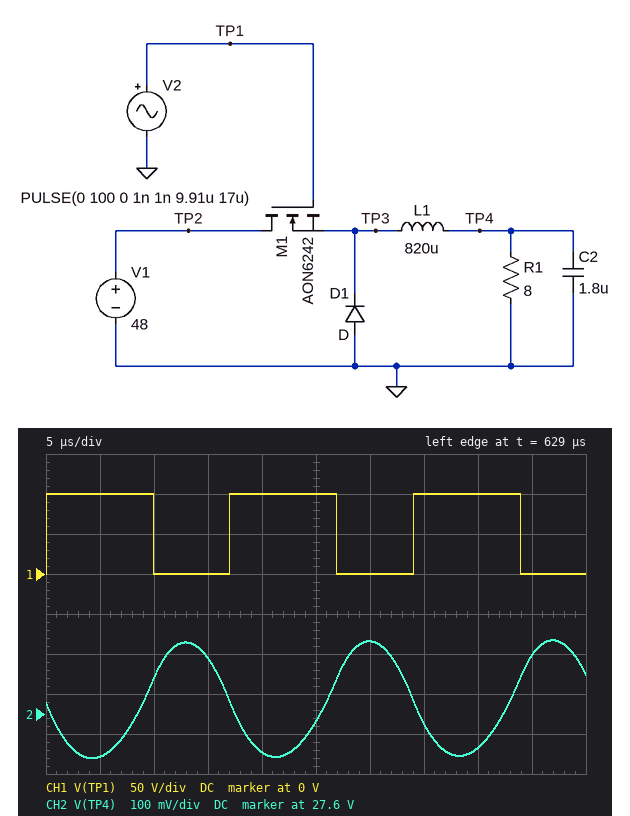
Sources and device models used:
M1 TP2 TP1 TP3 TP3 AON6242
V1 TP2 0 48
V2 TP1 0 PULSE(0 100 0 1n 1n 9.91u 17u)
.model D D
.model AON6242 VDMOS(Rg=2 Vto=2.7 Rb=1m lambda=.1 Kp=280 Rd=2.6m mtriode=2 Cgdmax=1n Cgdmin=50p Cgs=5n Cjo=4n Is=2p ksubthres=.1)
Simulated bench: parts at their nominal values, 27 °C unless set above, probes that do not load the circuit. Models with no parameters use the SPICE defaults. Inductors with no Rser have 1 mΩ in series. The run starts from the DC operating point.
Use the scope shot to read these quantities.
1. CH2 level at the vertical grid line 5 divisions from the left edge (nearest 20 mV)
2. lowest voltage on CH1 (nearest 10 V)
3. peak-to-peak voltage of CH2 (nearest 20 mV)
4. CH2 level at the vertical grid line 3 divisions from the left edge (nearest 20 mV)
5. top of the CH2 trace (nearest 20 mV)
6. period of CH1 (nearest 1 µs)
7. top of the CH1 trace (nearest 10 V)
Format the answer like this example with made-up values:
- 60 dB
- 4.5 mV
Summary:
- 27.58 V
- 0 V
- 300 mV
- 27.74 V
- 27.78 V
- 17 µs
- 100 V
